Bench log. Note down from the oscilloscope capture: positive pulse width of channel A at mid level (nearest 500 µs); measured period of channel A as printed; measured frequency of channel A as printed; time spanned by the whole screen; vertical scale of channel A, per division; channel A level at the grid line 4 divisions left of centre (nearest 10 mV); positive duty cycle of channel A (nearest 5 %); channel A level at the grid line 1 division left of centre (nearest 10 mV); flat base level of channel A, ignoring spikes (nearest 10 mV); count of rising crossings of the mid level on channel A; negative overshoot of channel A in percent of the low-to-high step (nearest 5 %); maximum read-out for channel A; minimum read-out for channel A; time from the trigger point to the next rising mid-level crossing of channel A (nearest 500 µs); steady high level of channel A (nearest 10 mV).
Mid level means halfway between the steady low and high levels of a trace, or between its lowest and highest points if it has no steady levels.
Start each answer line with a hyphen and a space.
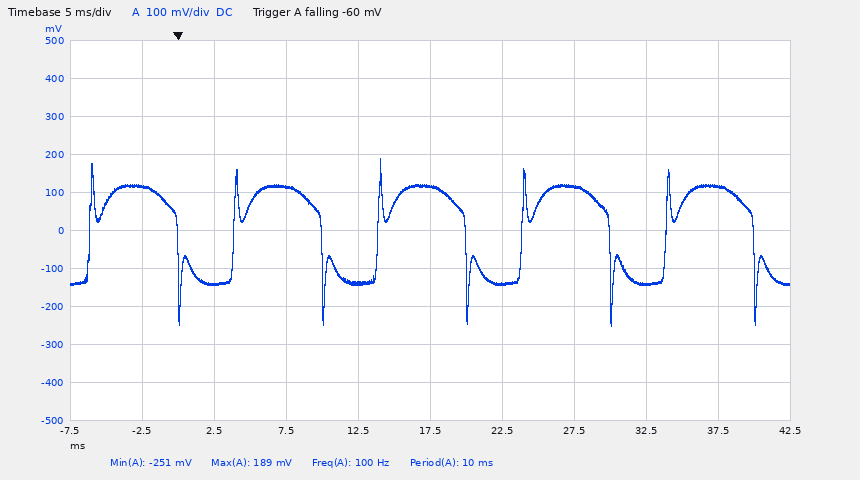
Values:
- 6.0 ms
- 10 ms
- 100 Hz
- 50 ms
- 100 mV
- 120 mV
- 60 %
- -140 mV
- -140 mV
- 5
- 45 %
- 189 mV
- -251 mV
- 4.0 ms
- 120 mV
